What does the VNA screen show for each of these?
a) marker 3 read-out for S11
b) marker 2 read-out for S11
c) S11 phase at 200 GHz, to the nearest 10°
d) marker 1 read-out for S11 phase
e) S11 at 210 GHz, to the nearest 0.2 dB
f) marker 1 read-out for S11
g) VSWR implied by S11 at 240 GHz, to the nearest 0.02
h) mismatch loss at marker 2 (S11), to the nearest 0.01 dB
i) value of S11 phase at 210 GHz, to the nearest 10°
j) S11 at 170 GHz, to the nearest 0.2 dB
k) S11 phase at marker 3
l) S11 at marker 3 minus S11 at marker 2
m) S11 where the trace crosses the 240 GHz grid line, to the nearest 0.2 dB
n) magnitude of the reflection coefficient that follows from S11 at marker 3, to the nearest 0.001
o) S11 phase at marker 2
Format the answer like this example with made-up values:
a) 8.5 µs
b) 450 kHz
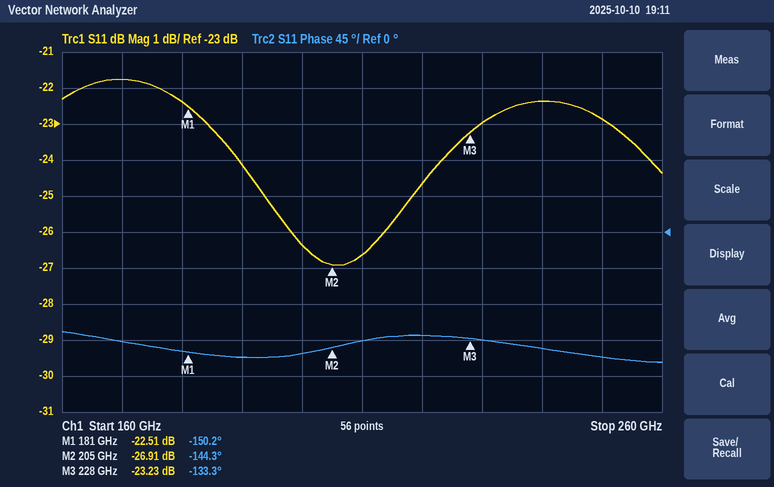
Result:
a) -23.23 dB
b) -26.91 dB
c) -150°
d) -150.2°
e) -26.6 dB
f) -22.51 dB
g) 1.16
h) 0.01 dB
i) -140°
j) -21.8 dB
k) -133.3°
l) 3.68 dB
m) -22.4 dB
n) 0.069
o) -144.3°
